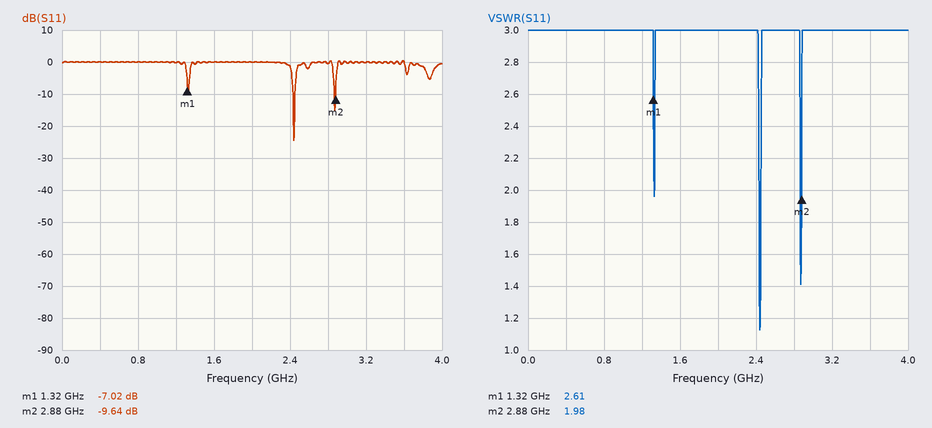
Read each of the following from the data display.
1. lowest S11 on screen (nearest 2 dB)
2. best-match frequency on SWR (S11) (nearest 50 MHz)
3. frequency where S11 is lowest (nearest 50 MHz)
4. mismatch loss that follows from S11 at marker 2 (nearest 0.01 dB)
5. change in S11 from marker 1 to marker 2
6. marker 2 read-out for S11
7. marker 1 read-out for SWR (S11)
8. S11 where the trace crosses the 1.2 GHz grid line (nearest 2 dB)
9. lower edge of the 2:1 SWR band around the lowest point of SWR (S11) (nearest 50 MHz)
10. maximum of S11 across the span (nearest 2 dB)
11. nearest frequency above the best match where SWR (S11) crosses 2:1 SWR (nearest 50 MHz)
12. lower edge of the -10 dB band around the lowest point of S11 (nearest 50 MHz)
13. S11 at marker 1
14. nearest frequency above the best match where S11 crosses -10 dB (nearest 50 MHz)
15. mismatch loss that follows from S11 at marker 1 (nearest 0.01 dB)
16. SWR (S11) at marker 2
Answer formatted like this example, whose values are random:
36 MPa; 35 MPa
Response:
-24 dB; 2.45 GHz; 2.45 GHz; 0.50 dB; -2.62 dB; -9.64 dB; 2.61; 0 dB; 2.45 GHz; 0 dB; 2.45 GHz; 2.45 GHz; -7.02 dB; 2.45 GHz; 0.96 dB; 1.98
